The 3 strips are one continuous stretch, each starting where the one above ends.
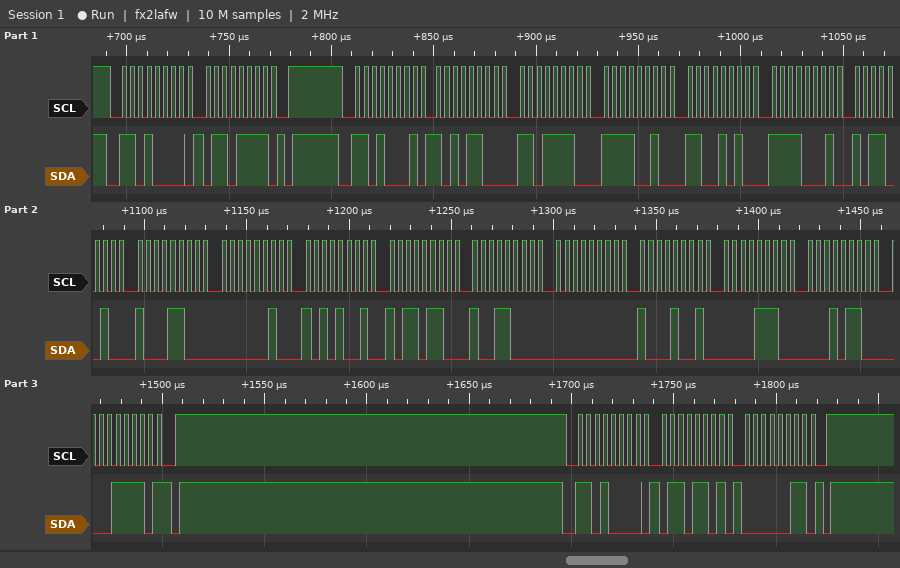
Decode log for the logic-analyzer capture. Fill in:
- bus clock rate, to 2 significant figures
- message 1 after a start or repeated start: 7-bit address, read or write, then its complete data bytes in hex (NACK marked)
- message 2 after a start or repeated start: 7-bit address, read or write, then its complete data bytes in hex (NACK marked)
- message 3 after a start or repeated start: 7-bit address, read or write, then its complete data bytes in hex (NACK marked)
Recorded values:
250 kHz
0x68 write: 6F
0x68 read: AC DE F2 CA F1 B2 8C 02 A9 B6 98 00 89 0E 16 1E NACK
0x68 write: 6D 03
